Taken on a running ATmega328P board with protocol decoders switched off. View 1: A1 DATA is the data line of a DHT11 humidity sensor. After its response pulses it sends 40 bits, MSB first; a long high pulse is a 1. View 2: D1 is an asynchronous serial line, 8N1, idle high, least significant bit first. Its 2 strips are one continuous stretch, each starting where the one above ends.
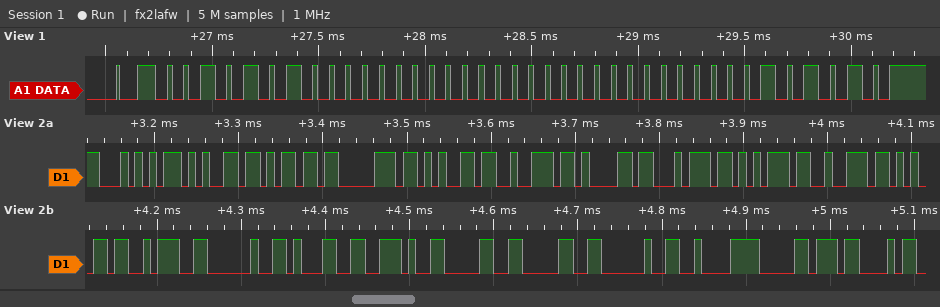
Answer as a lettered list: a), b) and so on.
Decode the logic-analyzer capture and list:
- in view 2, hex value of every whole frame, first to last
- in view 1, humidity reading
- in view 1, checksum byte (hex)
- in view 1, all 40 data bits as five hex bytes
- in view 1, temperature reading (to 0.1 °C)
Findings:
a) 54 65 6D 70 65 72 61 74 75 72 65 3A 20 31 2E 30 30 20 C2 B0 43
b) 42 %
c) 0x2A
d) 2A 00 00 00 2A
e) 0.0 °C
